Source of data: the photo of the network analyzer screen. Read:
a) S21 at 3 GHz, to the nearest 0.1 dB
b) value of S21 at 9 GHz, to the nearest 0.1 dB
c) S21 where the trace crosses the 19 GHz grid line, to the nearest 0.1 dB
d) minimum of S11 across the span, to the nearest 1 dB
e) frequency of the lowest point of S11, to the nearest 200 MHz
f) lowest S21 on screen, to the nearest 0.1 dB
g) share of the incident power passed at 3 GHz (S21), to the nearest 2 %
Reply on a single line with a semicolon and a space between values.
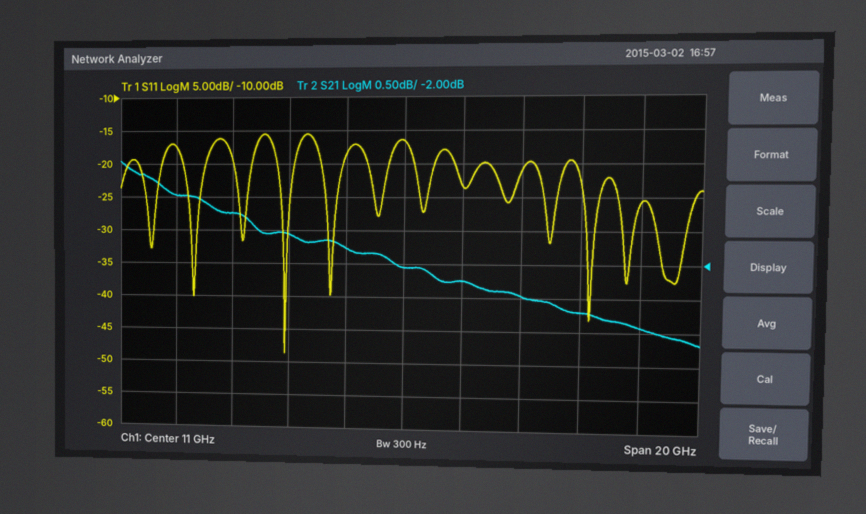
-1.0 dB; -1.8 dB; -2.9 dB; -49 dB; 6.8 GHz; -3.2 dB; 80 %
